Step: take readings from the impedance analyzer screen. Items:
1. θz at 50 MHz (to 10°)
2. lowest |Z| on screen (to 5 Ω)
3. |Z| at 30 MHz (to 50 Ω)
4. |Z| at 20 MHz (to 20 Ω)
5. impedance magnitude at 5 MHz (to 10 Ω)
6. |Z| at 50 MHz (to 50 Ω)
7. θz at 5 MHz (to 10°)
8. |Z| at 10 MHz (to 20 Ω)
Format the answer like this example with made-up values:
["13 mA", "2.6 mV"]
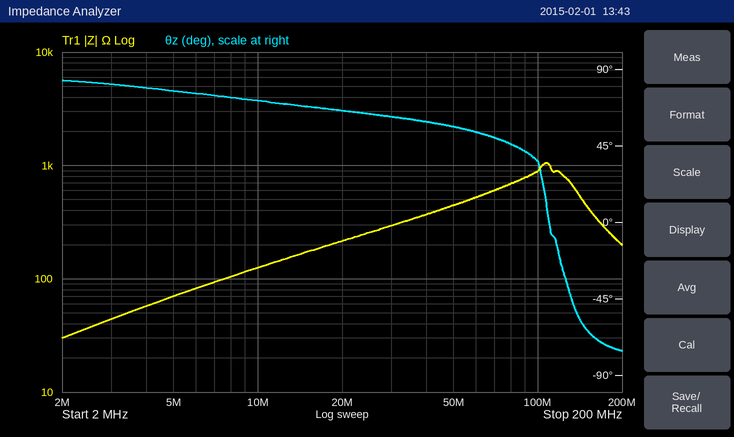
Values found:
["60°", "30 Ω", "300 Ω", "220 Ω", "70 Ω", "450 Ω", "80°", "120 Ω"]
